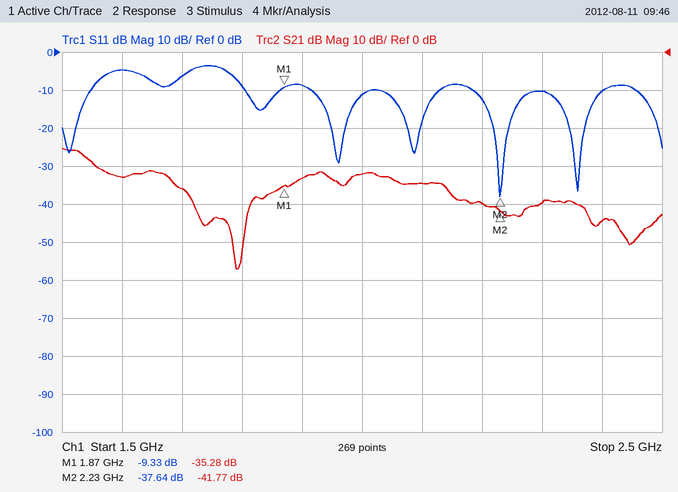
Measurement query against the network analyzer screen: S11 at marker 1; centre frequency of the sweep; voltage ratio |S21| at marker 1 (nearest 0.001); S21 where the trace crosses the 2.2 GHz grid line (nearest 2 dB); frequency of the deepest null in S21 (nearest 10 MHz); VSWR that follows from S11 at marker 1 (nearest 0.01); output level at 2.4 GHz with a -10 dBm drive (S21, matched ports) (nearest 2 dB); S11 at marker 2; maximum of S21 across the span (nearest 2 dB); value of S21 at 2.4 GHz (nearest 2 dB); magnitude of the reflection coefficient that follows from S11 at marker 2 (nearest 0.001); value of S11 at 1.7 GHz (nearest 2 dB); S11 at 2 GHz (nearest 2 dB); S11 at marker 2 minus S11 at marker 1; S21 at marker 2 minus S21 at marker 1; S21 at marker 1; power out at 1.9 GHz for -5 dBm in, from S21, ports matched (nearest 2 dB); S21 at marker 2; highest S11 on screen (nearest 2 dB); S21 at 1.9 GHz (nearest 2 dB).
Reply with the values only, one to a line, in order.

-9.33 dB
2 GHz
0.017
-40 dB
1.79 GHz
2.04
-54 dBm
-37.64 dB
-26 dB
-44 dB
0.013
-6 dB
-12 dB
-28.31 dB
-6.49 dB
-35.28 dB
-38 dBm
-41.77 dB
-4 dB
-34 dB
